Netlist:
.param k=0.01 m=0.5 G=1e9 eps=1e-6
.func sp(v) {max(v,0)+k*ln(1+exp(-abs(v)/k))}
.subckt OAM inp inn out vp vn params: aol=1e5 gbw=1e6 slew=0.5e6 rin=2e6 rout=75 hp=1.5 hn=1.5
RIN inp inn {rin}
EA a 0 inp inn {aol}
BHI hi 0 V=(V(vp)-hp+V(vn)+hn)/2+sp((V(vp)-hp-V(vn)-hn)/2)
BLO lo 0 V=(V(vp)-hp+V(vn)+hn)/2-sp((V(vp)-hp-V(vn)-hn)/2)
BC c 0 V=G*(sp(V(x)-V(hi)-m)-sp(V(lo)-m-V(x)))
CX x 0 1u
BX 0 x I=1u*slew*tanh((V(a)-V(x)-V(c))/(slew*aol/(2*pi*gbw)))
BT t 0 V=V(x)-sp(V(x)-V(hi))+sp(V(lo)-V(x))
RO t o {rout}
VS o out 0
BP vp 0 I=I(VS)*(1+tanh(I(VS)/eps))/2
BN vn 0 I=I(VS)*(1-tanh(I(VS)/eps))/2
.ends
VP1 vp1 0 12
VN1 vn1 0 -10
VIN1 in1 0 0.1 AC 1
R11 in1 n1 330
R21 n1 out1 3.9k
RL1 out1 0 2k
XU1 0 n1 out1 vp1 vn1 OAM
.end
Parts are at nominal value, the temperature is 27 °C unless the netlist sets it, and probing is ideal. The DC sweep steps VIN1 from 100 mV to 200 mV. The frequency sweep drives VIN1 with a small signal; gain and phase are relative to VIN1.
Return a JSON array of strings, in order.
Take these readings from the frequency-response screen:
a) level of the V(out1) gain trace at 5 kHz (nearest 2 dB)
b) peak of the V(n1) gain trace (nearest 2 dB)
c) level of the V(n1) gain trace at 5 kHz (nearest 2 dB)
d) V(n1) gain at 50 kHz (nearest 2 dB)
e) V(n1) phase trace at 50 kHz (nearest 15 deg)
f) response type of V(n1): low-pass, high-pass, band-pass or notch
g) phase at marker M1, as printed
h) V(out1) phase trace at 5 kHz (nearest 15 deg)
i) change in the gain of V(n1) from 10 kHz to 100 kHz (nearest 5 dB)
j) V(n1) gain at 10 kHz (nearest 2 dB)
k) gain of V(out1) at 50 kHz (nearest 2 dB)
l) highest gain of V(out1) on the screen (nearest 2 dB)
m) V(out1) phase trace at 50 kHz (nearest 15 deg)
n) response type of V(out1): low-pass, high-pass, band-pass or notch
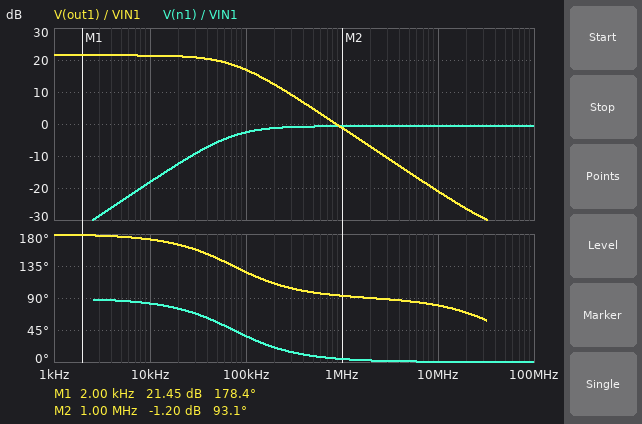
["22 dB", "0 dB", "-24 dB", "-6 dB", "60 deg", "high-pass", "178.4 deg", "180 deg", "15 dB", "-18 dB", "20 dB", "22 dB", "150 deg", "low-pass"]
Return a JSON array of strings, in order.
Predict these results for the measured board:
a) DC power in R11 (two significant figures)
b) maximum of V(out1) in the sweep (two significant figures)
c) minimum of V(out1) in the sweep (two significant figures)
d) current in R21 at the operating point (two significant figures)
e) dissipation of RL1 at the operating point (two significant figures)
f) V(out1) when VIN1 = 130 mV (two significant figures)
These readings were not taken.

["30 µW", "-1.2 V", "-2.4 V", "300 µA", "700 µW", "-1.5 V"]
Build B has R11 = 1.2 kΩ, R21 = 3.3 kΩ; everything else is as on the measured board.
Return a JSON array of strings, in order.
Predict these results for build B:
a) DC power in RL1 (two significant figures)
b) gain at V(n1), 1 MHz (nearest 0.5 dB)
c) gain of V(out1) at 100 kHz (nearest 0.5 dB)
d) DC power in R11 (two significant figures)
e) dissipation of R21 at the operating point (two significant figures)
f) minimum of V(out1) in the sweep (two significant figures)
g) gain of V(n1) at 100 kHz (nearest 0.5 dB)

["38 µW", "-3.0 dB", "8.0 dB", "8.3 µW", "23 µW", "-550 mV", "-11.5 dB"]
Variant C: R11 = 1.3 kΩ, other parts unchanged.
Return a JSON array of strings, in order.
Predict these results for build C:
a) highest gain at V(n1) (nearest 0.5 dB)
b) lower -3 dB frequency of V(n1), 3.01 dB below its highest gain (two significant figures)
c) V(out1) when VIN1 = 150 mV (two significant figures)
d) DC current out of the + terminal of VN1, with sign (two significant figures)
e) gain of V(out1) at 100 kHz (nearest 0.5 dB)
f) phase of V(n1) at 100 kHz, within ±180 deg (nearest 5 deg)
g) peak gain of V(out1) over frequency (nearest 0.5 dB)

["-2.5 dB", "240 kHz", "-450 mV", "-230 µA", "9.0 dB", "65 deg", "9.5 dB"]
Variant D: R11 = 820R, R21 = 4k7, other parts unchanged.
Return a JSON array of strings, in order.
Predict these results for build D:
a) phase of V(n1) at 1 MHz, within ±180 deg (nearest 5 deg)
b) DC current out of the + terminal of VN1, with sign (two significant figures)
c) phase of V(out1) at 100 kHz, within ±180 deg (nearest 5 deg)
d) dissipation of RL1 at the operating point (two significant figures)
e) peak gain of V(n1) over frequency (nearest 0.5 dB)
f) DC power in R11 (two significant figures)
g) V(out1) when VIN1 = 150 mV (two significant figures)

["10 deg", "-410 µA", "145 deg", "160 µW", "-1.5 dB", "12 µW", "-860 mV"]
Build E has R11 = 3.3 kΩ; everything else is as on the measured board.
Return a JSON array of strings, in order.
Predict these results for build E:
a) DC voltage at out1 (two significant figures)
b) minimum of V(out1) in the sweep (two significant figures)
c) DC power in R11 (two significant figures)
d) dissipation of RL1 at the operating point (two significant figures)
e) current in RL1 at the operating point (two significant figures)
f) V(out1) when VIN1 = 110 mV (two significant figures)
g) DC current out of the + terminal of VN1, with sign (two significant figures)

["-120 mV", "-240 mV", "3.0 µW", "7.0 µW", "59 µA", "-130 mV", "-89 µA"]
